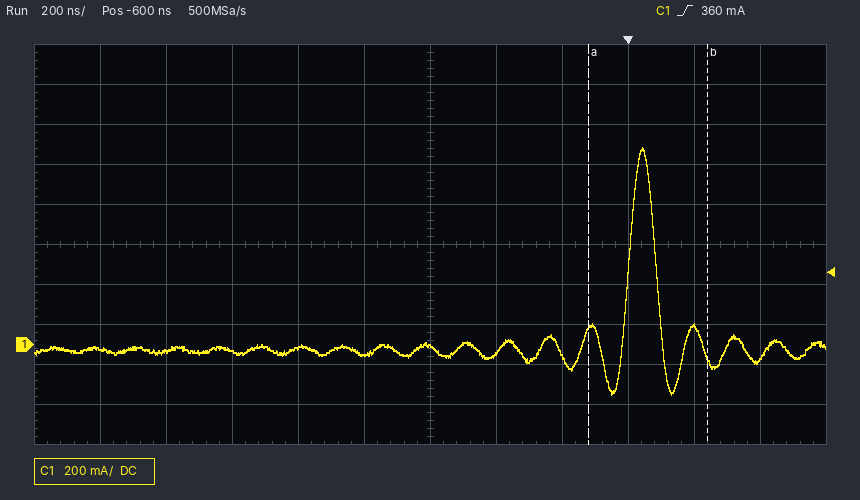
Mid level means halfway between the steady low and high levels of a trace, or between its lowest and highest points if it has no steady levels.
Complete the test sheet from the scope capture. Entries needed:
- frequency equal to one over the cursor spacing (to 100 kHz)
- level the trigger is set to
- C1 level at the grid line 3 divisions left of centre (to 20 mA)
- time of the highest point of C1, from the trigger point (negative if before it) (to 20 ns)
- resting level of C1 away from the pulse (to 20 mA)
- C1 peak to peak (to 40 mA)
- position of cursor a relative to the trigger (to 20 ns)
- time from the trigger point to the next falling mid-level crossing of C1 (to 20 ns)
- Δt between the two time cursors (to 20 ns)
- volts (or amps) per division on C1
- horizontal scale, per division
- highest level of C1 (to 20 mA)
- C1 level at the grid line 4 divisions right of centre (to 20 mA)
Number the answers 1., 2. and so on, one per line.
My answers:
1. 2.8 MHz
2. 360 mA
3. -40 mA
4. +40 ns
5. -20 mA
6. 1.24 A
7. -120 ns
8. 80 ns
9. 360 ns
10. 200 mA
11. 200 ns
12. 980 mA
13. 80 mA
